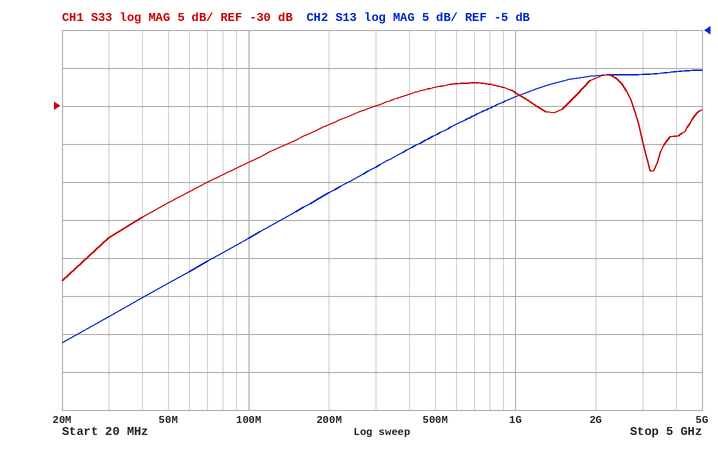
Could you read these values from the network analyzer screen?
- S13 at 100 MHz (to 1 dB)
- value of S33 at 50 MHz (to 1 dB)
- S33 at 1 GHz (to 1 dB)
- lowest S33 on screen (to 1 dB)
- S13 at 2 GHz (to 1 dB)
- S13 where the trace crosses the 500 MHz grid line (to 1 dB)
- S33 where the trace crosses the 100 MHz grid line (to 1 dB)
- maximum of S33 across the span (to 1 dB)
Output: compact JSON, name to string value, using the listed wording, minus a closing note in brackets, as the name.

{"S13 at 100 MHz": "-32 dB", "value of S33 at 50 MHz": "-43 dB", "S33 at 1 GHz": "-28 dB", "lowest S33 on screen": "-53 dB", "S13 at 2 GHz": "-11 dB", "S13 where the trace crosses the 500 MHz grid line": "-19 dB", "S33 where the trace crosses the 100 MHz grid line": "-37 dB", "maximum of S33 across the span": "-26 dB"}
